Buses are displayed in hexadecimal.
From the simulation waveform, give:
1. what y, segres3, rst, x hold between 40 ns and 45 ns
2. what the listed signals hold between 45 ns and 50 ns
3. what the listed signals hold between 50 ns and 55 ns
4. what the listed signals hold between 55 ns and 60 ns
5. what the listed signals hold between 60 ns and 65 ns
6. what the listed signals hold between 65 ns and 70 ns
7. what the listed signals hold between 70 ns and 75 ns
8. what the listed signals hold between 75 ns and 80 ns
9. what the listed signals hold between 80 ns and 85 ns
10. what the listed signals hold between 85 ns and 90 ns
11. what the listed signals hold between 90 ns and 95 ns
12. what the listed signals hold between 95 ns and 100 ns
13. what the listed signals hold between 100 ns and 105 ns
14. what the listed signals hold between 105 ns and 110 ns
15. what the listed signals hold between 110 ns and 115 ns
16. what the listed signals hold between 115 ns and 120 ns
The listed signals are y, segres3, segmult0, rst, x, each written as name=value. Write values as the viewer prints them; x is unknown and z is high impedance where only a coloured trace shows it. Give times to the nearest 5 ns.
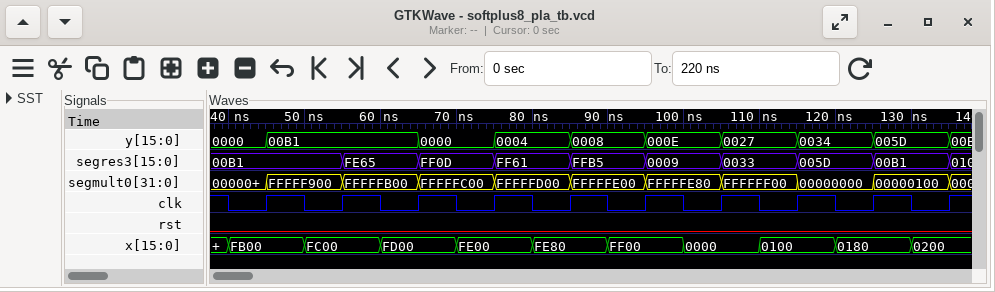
y=0000, segres3=00B1, rst=0, x=FB00
y=00B1, segres3=00B1, segmult0=FFFFF900, rst=0, x=FB00
y=00B1, segres3=00B1, segmult0=FFFFF900, rst=0, x=FC00
y=00B1, segres3=FE65, segmult0=FFFFFB00, rst=0, x=FC00
y=00B1, segres3=FE65, segmult0=FFFFFB00, rst=0, x=FD00
y=0000, segres3=FF0D, segmult0=FFFFFC00, rst=0, x=FD00
y=0000, segres3=FF0D, segmult0=FFFFFC00, rst=0, x=FE00
y=0004, segres3=FF61, segmult0=FFFFFD00, rst=0, x=FE00
y=0004, segres3=FF61, segmult0=FFFFFD00, rst=0, x=FE80
y=0008, segres3=FFB5, segmult0=FFFFFE00, rst=0, x=FE80
y=0008, segres3=FFB5, segmult0=FFFFFE00, rst=0, x=FF00
y=000E, segres3=0009, segmult0=FFFFFE80, rst=0, x=FF00
y=000E, segres3=0009, segmult0=FFFFFE80, rst=0, x=0000
y=0027, segres3=0033, segmult0=FFFFFF00, rst=0, x=0000
y=0027, segres3=0033, segmult0=FFFFFF00, rst=0, x=0100
y=0034, segres3=005D, segmult0=00000000, rst=0, x=0100
